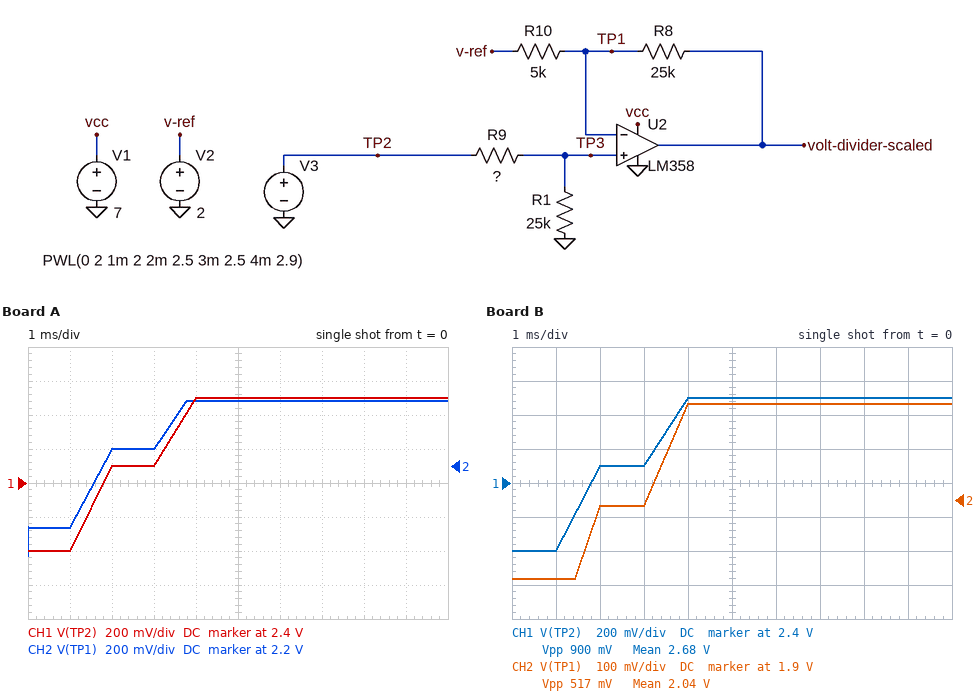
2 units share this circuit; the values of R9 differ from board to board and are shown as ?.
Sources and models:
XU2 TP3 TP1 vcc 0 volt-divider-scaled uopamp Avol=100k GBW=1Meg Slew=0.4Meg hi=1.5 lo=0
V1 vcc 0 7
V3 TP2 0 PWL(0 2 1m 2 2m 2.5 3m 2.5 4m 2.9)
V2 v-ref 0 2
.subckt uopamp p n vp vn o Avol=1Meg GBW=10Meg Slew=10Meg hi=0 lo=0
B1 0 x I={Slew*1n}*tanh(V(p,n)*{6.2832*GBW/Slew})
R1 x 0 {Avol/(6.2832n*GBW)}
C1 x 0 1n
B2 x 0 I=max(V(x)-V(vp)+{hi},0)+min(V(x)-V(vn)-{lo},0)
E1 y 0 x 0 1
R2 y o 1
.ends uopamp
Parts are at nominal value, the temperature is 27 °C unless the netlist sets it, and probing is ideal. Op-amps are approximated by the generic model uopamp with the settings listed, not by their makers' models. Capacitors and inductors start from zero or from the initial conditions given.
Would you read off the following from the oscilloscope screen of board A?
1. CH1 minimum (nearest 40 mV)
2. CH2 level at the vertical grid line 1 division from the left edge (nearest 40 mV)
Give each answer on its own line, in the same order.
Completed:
2.00 V
1.84 V
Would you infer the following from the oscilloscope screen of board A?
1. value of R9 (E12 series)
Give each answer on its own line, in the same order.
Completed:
2.2 kΩ
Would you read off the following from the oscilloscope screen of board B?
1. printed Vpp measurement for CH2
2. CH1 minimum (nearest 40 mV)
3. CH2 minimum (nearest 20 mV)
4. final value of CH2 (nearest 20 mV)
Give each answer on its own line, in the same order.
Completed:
517 mV
2.00 V
1.66 V
2.18 V
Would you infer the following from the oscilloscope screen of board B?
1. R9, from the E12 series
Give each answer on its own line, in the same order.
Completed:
8.2 kΩ
